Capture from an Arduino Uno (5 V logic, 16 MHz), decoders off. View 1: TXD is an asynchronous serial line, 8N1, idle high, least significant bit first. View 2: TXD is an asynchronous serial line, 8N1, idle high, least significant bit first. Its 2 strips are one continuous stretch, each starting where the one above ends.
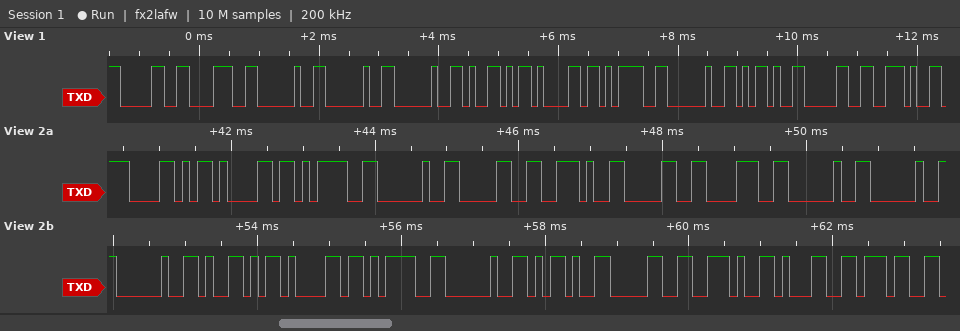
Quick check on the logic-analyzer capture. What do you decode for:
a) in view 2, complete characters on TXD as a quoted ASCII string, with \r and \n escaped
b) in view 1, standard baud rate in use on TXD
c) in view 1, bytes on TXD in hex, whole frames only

"Xa= 0.08   Ya= -0.17"
9600 baud
0x30 0x38 0x20 0x20 0x20 0x59 0x61 0x3D 0x20 0x2D 0x30 0x2E
